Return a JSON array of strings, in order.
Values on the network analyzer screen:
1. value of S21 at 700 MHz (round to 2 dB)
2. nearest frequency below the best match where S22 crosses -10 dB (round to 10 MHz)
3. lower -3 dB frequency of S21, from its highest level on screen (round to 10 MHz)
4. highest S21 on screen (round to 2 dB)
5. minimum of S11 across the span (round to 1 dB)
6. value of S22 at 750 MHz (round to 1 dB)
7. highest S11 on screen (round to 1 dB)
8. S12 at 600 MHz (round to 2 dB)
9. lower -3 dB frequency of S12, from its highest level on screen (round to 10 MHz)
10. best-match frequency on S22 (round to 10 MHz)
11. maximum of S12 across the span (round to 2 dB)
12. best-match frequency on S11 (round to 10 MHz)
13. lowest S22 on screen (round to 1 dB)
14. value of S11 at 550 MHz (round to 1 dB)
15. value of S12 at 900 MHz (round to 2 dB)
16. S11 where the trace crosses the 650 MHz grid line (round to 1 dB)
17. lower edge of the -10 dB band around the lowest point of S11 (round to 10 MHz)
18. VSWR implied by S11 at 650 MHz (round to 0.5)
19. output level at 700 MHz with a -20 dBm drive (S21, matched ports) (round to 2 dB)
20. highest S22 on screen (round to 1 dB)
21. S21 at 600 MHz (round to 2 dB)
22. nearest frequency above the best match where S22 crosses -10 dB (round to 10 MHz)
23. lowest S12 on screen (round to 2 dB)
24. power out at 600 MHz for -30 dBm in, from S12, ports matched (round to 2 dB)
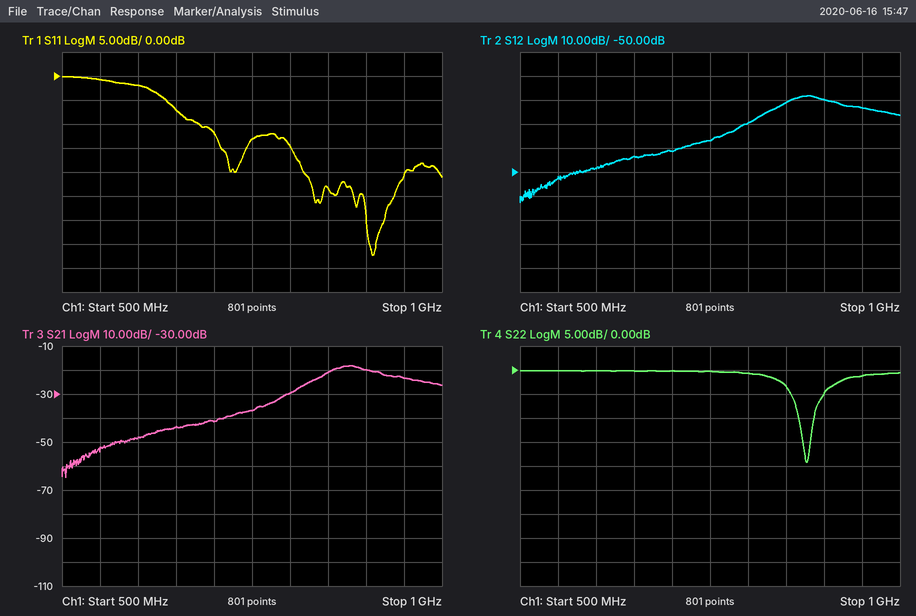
["-42 dB", "870 MHz", "850 MHz", "-18 dB", "-37 dB", "0 dB", "0 dB", "-48 dB", "850 MHz", "880 MHz", "-18 dB", "910 MHz", "-19 dB", "-1 dB", "-20 dB", "-7 dB", "680 MHz", "2.5", "-62 dBm", "0 dB", "-48 dB", "890 MHz", "-62 dB", "-78 dBm"]
